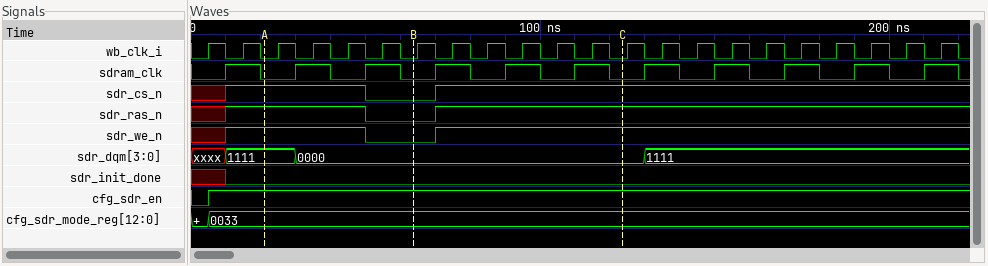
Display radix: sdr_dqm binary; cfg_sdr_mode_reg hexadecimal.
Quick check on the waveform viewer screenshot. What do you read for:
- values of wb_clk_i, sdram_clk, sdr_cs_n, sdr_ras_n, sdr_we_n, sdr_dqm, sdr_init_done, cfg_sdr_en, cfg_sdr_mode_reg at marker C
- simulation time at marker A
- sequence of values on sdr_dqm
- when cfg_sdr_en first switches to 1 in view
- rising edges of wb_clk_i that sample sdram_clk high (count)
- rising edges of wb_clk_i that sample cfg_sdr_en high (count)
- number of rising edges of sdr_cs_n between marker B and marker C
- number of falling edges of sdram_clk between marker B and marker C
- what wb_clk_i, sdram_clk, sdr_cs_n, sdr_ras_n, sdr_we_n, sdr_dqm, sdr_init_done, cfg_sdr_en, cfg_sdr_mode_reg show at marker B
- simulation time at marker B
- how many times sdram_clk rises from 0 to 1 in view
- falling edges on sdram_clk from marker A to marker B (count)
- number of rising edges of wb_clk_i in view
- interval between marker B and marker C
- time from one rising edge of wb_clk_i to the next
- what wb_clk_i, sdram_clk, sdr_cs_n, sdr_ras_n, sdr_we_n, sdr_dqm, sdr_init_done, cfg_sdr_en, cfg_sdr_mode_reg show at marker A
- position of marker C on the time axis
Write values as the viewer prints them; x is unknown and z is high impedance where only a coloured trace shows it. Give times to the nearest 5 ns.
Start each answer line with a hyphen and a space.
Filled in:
- wb_clk_i=0, sdram_clk=0, sdr_cs_n=1, sdr_ras_n=1, sdr_we_n=1, sdr_dqm=0000, sdr_init_done=0, cfg_sdr_en=1, cfg_sdr_mode_reg=0033
- 20 ns
- xxxx, 1111, 0000, 1111
- 5 ns
- 11
- 21
- 1
- 3
- wb_clk_i=0, sdram_clk=0, sdr_cs_n=0, sdr_ras_n=0, sdr_we_n=0, sdr_dqm=0000, sdr_init_done=0, cfg_sdr_en=1, cfg_sdr_mode_reg=0033
- 65 ns
- 11
- 2
- 22
- 60 ns
- 10 ns
- wb_clk_i=0, sdram_clk=0, sdr_cs_n=1, sdr_ras_n=1, sdr_we_n=1, sdr_dqm=1111, sdr_init_done=0, cfg_sdr_en=1, cfg_sdr_mode_reg=0033
- 125 ns
